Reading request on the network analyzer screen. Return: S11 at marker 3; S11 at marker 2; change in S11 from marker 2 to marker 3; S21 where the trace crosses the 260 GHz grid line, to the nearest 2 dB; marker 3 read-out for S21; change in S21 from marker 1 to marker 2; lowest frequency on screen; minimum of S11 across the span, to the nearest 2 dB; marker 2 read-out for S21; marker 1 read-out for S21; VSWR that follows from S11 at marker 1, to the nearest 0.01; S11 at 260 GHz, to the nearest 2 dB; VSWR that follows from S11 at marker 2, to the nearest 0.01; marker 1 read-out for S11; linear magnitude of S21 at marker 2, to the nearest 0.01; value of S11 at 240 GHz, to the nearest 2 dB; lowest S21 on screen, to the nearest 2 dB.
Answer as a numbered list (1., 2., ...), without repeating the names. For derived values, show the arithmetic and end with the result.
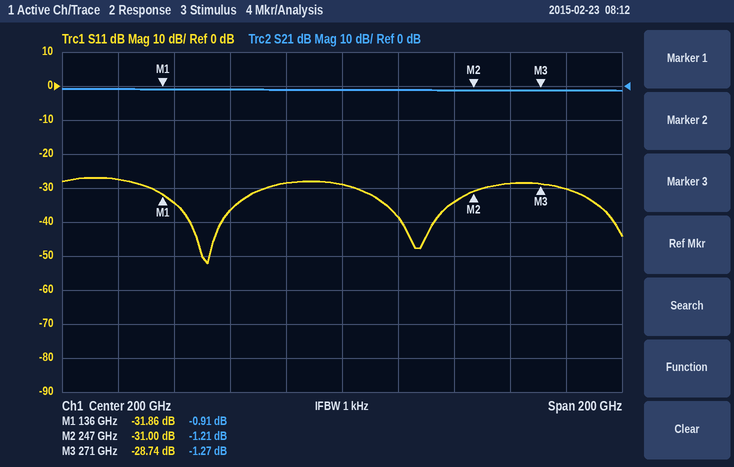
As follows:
1. -28.74 dB
2. -31.00 dB
3. -28.74 − (-31) = 2.26 dB
4. -2 dB
5. -1.27 dB
6. -1.21 − (-0.91) = -0.30 dB
7. 100 GHz
8. -52 dB
9. -1.21 dB
10. -0.91 dB
11. (1 + 0.0255)/(1 − 0.0255) ≈ 1.05
12. -28 dB
13. (1 + 0.0282)/(1 − 0.0282) ≈ 1.06
14. -31.86 dB
15. 10^(-1.21/20) ≈ 0.87
16. -34 dB
17. -2 dB
